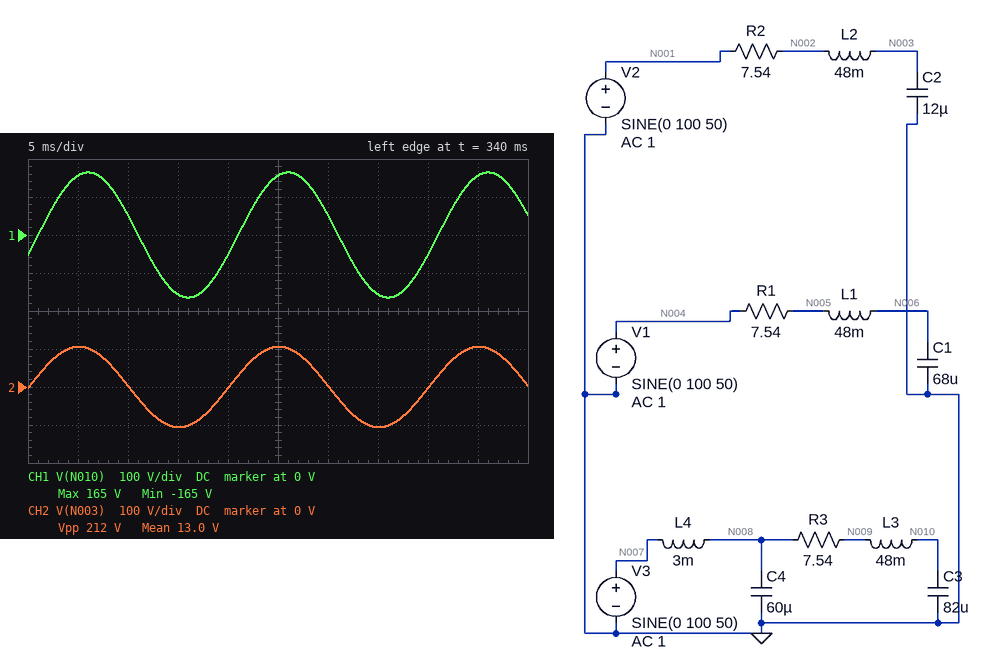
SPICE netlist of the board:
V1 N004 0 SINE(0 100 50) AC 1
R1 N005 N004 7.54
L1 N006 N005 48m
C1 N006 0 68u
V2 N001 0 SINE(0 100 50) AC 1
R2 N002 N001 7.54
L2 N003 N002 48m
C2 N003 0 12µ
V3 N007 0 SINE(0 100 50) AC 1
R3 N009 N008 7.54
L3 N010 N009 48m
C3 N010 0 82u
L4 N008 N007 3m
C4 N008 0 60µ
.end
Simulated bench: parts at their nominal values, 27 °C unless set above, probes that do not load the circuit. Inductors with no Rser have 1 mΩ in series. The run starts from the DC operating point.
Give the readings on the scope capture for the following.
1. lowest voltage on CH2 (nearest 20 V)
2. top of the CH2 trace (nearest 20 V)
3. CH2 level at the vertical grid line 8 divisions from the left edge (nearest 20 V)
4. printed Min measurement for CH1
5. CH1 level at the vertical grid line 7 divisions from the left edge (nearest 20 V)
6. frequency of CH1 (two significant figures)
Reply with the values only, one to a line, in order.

-100 V
100 V
0 V
-165 V
-160 V
50 Hz
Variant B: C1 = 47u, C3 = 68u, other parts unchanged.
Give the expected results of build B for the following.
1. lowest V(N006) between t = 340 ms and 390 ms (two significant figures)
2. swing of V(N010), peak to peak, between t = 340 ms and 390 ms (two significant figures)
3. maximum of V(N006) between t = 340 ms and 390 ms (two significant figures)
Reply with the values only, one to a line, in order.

-130 V
300 V
130 V
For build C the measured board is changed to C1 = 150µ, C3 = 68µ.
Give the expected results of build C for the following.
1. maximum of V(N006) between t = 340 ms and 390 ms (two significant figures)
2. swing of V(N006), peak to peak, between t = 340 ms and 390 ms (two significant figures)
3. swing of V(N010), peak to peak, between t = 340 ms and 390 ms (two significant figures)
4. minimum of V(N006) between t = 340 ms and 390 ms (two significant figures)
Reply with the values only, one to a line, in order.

220 V
440 V
300 V
-220 V
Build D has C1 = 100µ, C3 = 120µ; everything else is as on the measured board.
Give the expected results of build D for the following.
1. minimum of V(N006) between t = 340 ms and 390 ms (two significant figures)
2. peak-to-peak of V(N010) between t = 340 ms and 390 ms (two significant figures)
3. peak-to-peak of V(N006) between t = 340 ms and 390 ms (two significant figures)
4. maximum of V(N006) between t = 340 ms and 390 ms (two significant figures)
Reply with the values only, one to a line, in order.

-170 V
420 V
350 V
170 V
